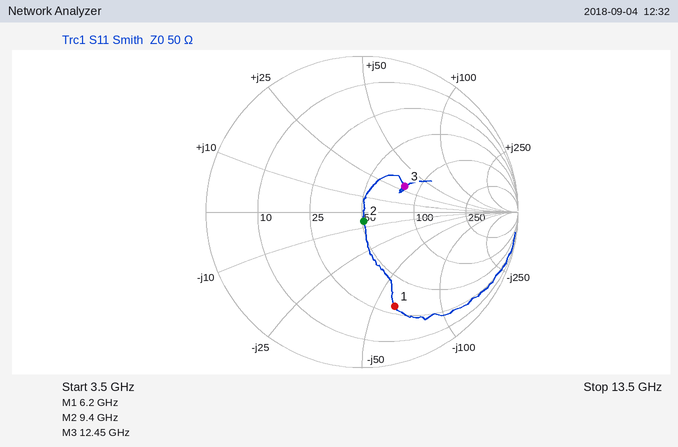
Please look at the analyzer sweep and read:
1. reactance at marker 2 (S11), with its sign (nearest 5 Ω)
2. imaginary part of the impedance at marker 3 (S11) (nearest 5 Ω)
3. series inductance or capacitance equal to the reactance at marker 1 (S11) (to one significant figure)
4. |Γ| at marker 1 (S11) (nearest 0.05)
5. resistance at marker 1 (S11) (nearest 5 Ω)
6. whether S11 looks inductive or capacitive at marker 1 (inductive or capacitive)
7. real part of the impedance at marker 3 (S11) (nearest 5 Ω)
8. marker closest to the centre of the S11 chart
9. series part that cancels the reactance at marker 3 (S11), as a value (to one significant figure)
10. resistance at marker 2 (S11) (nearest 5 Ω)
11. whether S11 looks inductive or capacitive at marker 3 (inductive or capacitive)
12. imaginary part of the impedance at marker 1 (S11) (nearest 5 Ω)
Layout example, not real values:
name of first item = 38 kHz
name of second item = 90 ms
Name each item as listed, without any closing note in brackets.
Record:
reactance at marker 2 (S11), with its sign = -5 Ω
imaginary part of the impedance at marker 3 (S11) = +30 Ω
series inductance or capacitance equal to the reactance at marker 1 (S11) = 400 fF
|Γ| at marker 1 (S11) = 0.65
resistance at marker 1 (S11) = 30 Ω
whether S11 looks inductive or capacitive at marker 1 = capacitive
real part of the impedance at marker 3 (S11) = 80 Ω
marker closest to the centre of the S11 chart = marker 2
series part that cancels the reactance at marker 3 (S11), as a value = 400 fF
resistance at marker 2 (S11) = 50 Ω
whether S11 looks inductive or capacitive at marker 3 = inductive
imaginary part of the impedance at marker 1 (S11) = -60 Ω
